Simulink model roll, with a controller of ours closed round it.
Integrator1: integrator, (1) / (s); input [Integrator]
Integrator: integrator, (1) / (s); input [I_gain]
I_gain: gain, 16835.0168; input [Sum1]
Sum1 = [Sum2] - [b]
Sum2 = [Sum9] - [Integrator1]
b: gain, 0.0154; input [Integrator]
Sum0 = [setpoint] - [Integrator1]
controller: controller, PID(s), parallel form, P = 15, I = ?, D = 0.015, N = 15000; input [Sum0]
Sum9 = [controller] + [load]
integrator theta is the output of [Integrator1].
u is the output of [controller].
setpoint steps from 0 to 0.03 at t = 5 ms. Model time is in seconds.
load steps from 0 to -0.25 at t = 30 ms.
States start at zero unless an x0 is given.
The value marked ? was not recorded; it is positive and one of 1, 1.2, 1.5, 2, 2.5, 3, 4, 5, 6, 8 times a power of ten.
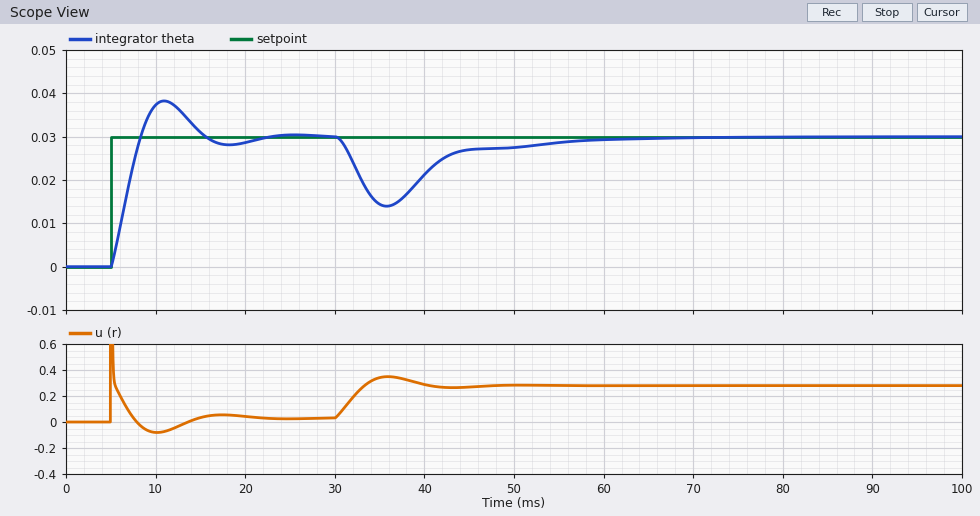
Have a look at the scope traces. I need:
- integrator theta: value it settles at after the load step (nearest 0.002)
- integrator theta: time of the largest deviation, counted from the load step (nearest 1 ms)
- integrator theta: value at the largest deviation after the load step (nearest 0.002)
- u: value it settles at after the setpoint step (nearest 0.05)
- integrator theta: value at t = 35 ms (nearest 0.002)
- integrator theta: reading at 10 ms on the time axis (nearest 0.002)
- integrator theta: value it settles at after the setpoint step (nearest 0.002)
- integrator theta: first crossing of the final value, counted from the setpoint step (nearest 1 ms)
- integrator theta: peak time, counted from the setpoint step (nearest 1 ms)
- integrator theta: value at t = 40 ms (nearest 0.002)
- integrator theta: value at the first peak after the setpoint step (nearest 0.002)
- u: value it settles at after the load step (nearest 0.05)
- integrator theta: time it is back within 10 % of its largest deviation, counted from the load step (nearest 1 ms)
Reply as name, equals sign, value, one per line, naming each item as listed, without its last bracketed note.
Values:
integrator theta: value it settles at after the load step = 0.030
integrator theta: time of the largest deviation, counted from the load step = 6 ms
integrator theta: value at the largest deviation after the load step = 0.014
u: value it settles at after the setpoint step = 0.05
integrator theta: value at t = 35 ms = 0.014
integrator theta: reading at 10 ms on the time axis = 0.038
integrator theta: value it settles at after the setpoint step = 0.030
integrator theta: first crossing of the final value, counted from the setpoint step = 3 ms
integrator theta: peak time, counted from the setpoint step = 6 ms
integrator theta: value at t = 40 ms = 0.022
integrator theta: value at the first peak after the setpoint step = 0.038
u: value it settles at after the load step = 0.30
integrator theta: time it is back within 10 % of its largest deviation, counted from the load step = 24 ms
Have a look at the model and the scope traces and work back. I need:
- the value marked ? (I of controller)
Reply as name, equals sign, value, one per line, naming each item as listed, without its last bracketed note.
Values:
the value marked ? = 1500
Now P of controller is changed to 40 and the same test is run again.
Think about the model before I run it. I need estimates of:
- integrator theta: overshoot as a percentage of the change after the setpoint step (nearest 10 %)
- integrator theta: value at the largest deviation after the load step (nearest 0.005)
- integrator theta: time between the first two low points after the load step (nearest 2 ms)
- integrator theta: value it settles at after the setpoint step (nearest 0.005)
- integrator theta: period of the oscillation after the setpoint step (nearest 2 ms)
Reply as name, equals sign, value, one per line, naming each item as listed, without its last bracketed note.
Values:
integrator theta: overshoot as a percentage of the change after the setpoint step = 40 %
integrator theta: value at the largest deviation after the load step = 0.020
integrator theta: time between the first two low points after the load step = 8 ms
integrator theta: value it settles at after the setpoint step = 0.030
integrator theta: period of the oscillation after the setpoint step = 8 ms
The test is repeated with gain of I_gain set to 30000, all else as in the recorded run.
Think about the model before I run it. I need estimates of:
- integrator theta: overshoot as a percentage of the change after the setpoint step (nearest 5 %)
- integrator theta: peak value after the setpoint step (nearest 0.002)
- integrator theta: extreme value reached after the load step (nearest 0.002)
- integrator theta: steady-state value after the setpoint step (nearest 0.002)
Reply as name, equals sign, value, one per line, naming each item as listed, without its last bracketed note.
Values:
integrator theta: overshoot as a percentage of the change after the setpoint step = 15 %
integrator theta: peak value after the setpoint step = 0.034
integrator theta: extreme value reached after the load step = 0.016
integrator theta: steady-state value after the setpoint step = 0.030
